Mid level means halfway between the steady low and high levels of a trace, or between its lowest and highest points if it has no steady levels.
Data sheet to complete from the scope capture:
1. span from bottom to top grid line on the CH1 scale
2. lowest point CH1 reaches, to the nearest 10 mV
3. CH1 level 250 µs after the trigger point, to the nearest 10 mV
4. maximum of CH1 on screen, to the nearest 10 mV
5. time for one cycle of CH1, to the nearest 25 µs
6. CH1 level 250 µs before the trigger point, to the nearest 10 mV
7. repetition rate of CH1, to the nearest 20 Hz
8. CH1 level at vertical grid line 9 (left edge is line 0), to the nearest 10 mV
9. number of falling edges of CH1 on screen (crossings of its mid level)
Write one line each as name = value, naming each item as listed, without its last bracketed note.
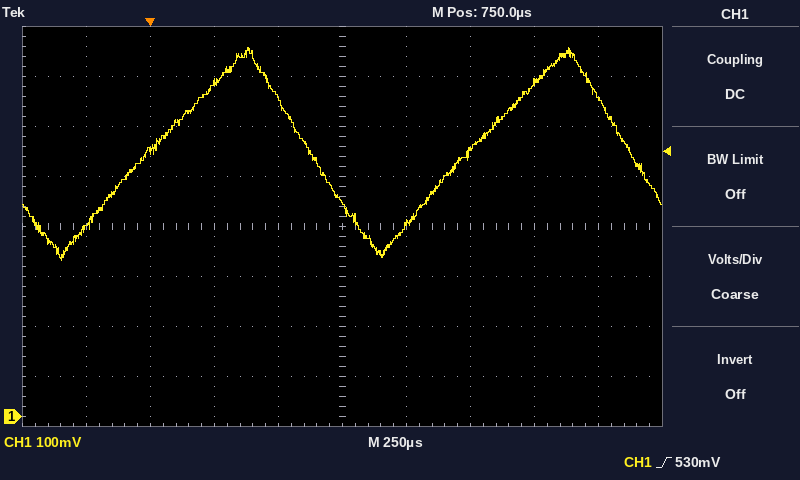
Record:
span from bottom to top grid line on the CH1 scale = 800 mV
lowest point CH1 reaches, to the nearest 10 mV = 310 mV
CH1 level 250 µs after the trigger point, to the nearest 10 mV = 670 mV
maximum of CH1 on screen, to the nearest 10 mV = 740 mV
time for one cycle of CH1, to the nearest 25 µs = 1.250 ms
CH1 level 250 µs before the trigger point, to the nearest 10 mV = 380 mV
repetition rate of CH1, to the nearest 20 Hz = 800 Hz
CH1 level at vertical grid line 9 (left edge is line 0), to the nearest 10 mV = 640 mV
number of falling edges of CH1 on screen = 2
